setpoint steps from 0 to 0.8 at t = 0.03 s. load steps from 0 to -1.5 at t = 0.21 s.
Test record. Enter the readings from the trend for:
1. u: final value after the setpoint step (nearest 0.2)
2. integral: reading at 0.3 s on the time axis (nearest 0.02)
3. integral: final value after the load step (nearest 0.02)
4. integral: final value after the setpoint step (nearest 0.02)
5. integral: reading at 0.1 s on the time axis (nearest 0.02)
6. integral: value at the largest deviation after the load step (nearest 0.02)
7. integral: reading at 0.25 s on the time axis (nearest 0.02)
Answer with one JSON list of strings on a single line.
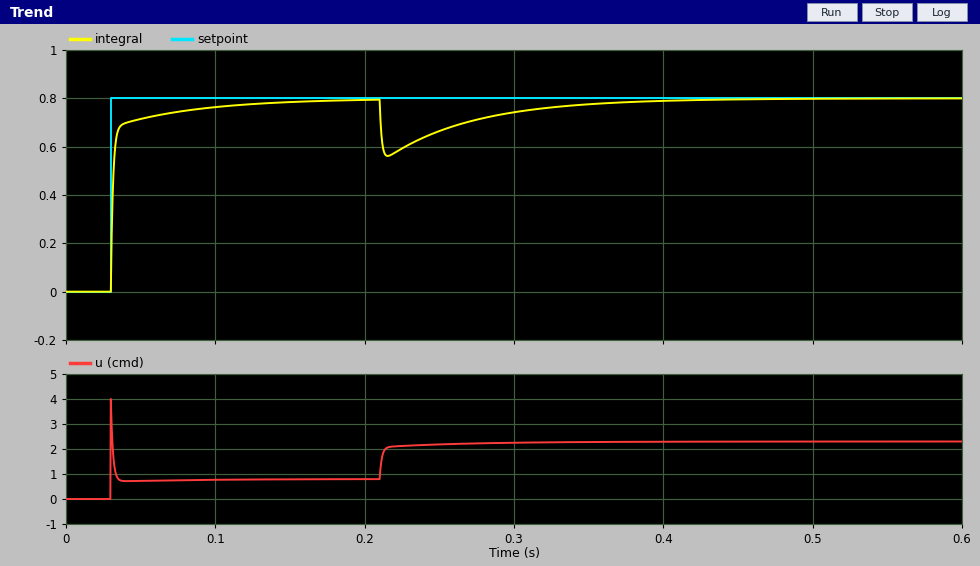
["0.8", "0.74", "0.80", "0.80", "0.76", "0.56", "0.66"]
